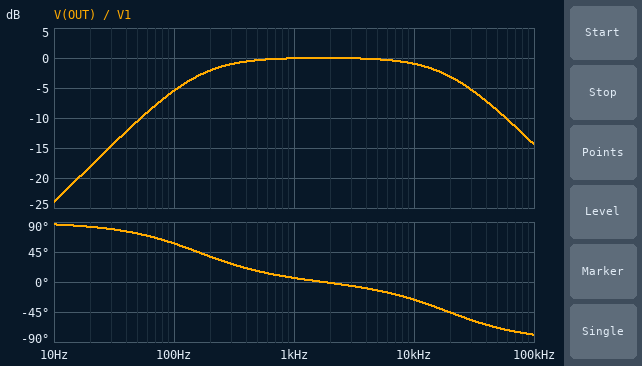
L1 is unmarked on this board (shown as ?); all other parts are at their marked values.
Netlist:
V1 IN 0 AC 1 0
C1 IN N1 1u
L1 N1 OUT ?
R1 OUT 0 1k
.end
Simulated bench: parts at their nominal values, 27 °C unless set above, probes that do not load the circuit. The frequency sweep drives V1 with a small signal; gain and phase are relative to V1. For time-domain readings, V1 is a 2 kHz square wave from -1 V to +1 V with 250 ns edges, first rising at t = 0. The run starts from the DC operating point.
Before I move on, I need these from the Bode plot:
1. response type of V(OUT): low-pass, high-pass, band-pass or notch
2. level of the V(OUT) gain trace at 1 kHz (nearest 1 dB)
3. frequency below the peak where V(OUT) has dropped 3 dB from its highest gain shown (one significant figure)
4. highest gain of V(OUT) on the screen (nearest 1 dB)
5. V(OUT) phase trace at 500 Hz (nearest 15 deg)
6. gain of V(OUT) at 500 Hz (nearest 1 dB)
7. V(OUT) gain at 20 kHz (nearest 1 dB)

band-pass
0 dB
200 Hz
0 dB
15 deg
0 dB
-3 dB
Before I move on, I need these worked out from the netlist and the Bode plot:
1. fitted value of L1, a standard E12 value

8.2 mH
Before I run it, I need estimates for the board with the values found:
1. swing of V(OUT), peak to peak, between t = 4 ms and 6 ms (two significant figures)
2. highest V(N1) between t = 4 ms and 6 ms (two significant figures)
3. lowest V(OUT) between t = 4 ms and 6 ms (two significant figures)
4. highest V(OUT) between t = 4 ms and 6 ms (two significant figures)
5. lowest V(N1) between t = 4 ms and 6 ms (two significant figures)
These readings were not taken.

2.2 V
1.1 V
-1.1 V
1.1 V
-1.1 V
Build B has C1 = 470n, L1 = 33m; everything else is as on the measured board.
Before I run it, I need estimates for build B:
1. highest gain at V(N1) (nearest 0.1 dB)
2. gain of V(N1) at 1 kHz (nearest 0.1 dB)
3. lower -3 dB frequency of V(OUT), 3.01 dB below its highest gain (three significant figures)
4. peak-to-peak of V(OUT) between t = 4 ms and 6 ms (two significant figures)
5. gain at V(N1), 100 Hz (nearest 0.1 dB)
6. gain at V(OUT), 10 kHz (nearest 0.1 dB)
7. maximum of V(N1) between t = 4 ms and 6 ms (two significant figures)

0.4 dB
0.1 dB
318 Hz
2.1 V
-10.9 dB
-7.1 dB
1.2 V
